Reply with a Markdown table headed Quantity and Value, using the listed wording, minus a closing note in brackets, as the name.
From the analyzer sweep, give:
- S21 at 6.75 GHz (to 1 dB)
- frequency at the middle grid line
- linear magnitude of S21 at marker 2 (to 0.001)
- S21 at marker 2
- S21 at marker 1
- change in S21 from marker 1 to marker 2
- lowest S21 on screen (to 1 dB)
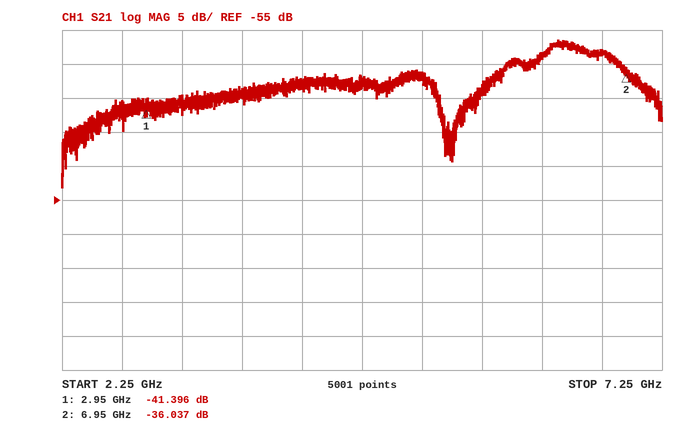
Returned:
| Quantity | Value |
|---|---|
| S21 at 6.75 GHz | -33 dB |
| frequency at the middle grid line | 4.75 GHz |
| linear magnitude of S21 at marker 2 | 0.016 |
| S21 at marker 2 | -36.037 dB |
| S21 at marker 1 | -41.396 dB |
| change in S21 from marker 1 to marker 2 | 5.359 dB |
| lowest S21 on screen | -53 dB |
